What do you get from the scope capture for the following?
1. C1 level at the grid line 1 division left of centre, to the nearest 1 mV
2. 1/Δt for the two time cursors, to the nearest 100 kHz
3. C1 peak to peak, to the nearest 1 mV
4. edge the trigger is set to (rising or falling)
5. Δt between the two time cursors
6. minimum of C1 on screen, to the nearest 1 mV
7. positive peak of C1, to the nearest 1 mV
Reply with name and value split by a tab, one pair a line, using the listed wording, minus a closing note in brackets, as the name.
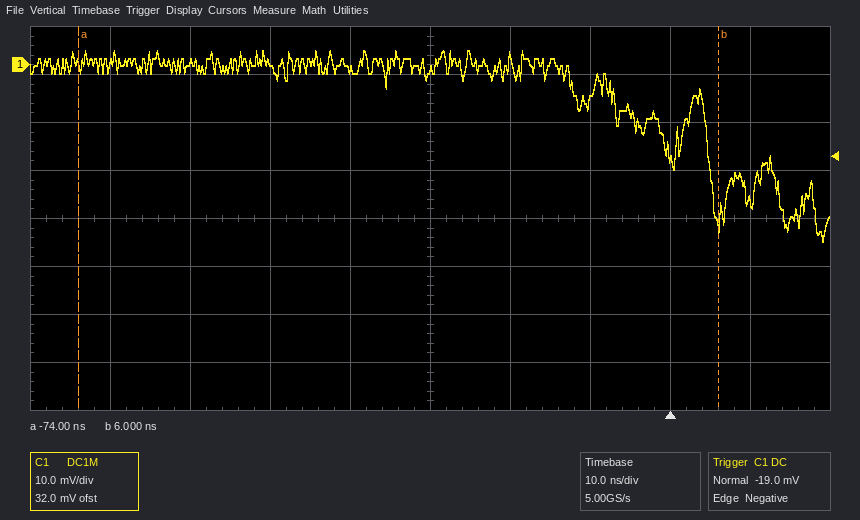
C1 level at the grid line 1 division left of centre, to the nearest 1 mV	-1 mV
1/Δt for the two time cursors, to the nearest 100 kHz	12.5 MHz
C1 peak to peak, to the nearest 1 mV	40 mV
edge the trigger is set to	falling
Δt between the two time cursors	80 ns
minimum of C1 on screen, to the nearest 1 mV	-37 mV
positive peak of C1, to the nearest 1 mV	3 mV
